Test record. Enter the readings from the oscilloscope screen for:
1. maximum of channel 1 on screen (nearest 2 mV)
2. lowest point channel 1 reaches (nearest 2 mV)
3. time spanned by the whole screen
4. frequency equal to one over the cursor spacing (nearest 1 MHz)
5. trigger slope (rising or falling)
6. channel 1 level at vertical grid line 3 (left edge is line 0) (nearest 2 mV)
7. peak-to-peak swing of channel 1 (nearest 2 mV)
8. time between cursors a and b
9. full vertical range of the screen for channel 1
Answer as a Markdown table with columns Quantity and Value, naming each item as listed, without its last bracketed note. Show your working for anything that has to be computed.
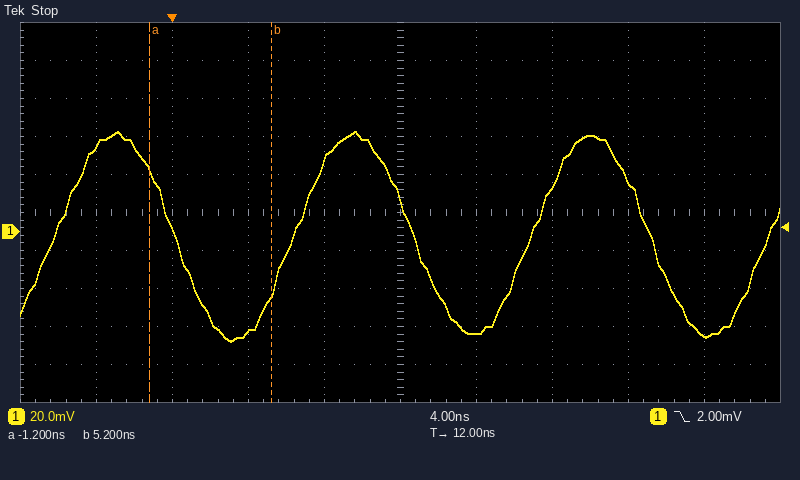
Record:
| Quantity | Value |
|---|---|
| maximum of channel 1 on screen | 52 mV |
| lowest point channel 1 reaches | -58 mV |
| time spanned by the whole screen | 40 ns |
| frequency equal to one over the cursor spacing | 1 / 6.4 ns ≈ 156 MHz |
| trigger slope | falling |
| channel 1 level at vertical grid line 3 (left edge is line 0) | -54 mV |
| peak-to-peak swing of channel 1 | 52 mV − (-58 mV) = 110 mV |
| time between cursors a and b | 5.2 ns − (-1.2 ns) = 6.4 ns |
| full vertical range of the screen for channel 1 | 200 mV |
